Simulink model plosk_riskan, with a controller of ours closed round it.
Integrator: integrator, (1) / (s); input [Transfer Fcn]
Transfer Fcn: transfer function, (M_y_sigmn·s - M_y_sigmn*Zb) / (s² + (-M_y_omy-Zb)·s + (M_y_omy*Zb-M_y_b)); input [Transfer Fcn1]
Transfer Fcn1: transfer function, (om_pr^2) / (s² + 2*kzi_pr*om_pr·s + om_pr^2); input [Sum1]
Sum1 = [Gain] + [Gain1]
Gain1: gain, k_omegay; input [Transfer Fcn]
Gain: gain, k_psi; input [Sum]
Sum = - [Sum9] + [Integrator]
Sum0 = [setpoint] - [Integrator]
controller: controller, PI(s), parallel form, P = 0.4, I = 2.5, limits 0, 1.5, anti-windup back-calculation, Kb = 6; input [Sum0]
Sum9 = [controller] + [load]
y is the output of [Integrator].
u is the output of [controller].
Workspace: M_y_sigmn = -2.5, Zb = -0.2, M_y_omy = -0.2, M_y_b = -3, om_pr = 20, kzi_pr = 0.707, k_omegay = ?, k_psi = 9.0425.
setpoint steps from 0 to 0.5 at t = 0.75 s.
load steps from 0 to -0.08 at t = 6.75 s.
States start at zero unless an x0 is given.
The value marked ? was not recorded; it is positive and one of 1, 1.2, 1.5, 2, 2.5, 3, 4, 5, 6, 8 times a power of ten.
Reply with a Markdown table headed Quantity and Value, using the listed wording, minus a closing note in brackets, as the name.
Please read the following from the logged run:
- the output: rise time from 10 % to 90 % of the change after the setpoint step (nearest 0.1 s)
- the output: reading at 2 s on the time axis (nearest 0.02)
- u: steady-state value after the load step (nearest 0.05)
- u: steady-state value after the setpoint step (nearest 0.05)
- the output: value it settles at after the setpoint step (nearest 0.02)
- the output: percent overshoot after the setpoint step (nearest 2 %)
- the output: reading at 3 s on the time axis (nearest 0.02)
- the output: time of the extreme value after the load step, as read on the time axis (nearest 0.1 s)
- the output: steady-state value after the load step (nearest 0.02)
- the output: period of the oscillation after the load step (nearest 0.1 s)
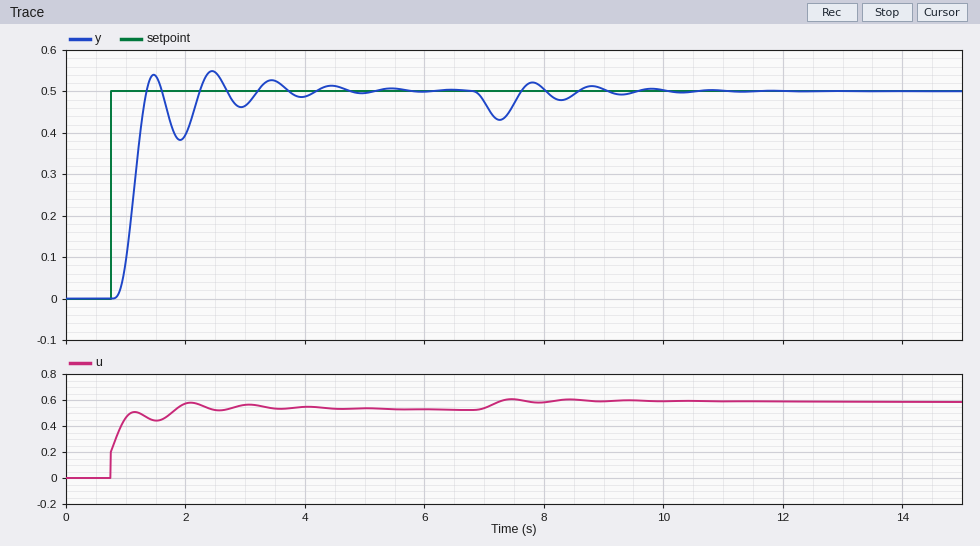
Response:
| Quantity | Value |
|---|---|
| the output: rise time from 10 % to 90 % of the change after the setpoint step | 0.3 s |
| the output: reading at 2 s on the time axis | 0.40 |
| u: steady-state value after the load step | 0.60 |
| u: steady-state value after the setpoint step | 0.50 |
| the output: value it settles at after the setpoint step | 0.50 |
| the output: percent overshoot after the setpoint step | 10 % |
| the output: reading at 3 s on the time axis | 0.46 |
| the output: time of the extreme value after the load step, as read on the time axis | 7.3 s |
| the output: steady-state value after the load step | 0.50 |
| the output: period of the oscillation after the load step | 1.0 s |
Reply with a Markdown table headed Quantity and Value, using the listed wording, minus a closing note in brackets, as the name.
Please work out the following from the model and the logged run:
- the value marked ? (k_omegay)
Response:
| Quantity | Value |
|---|---|
| the value marked ? | 2 |
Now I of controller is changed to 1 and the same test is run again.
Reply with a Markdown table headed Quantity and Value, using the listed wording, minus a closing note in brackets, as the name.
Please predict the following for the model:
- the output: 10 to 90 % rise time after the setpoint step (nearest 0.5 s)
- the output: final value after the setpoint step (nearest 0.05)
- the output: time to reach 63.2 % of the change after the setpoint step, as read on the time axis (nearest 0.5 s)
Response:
| Quantity | Value |
|---|---|
| the output: 10 to 90 % rise time after the setpoint step | 2.5 s |
| the output: final value after the setpoint step | 0.50 |
| the output: time to reach 63.2 % of the change after the setpoint step, as read on the time axis | 1.5 s |
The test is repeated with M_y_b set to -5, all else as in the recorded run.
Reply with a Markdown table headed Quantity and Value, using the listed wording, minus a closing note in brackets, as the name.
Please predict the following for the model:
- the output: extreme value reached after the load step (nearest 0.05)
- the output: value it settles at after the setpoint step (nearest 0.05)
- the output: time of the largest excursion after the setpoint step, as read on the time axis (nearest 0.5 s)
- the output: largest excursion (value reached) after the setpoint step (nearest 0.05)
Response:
| Quantity | Value |
|---|---|
| the output: extreme value reached after the load step | 0.45 |
| the output: value it settles at after the setpoint step | 0.50 |
| the output: time of the largest excursion after the setpoint step, as read on the time axis | 2.5 s |
| the output: largest excursion (value reached) after the setpoint step | 0.55 |
